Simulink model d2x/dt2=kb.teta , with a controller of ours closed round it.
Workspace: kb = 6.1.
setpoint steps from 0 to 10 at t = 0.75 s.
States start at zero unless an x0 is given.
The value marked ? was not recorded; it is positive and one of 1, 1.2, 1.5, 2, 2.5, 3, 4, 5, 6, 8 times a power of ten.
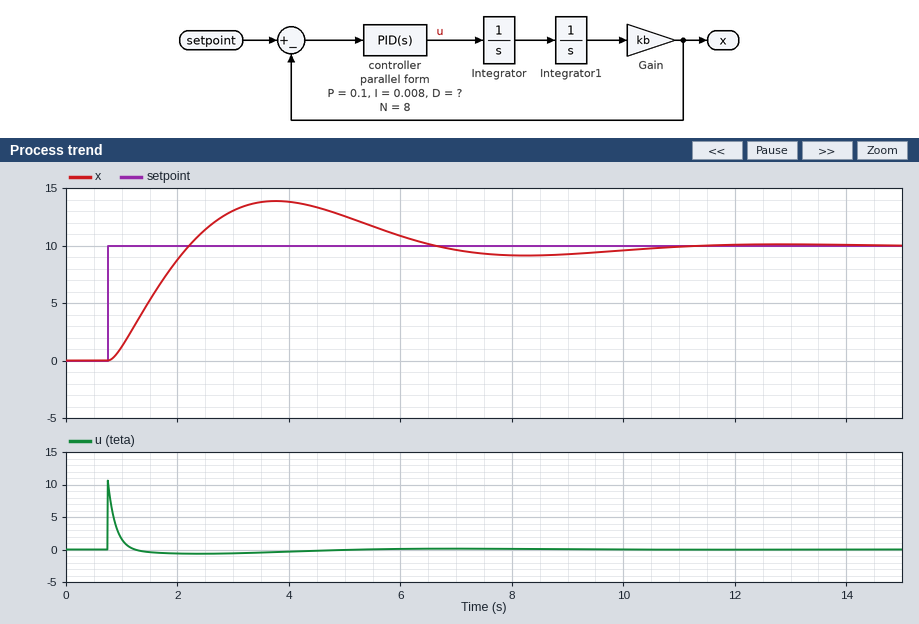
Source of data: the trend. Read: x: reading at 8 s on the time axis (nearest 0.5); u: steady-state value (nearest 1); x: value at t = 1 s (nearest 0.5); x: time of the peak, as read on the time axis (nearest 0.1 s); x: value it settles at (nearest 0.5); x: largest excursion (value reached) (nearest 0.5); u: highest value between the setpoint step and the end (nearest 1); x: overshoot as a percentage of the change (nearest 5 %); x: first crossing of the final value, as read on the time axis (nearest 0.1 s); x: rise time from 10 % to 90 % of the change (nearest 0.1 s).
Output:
9.0
0
1.0
3.8 s
10.0
14.0
11
40 %
2.2 s
1.1 s
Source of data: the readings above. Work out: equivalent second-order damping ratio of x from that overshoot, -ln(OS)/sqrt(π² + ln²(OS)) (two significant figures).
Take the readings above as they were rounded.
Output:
0.28
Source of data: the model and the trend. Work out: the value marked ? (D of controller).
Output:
0.12
